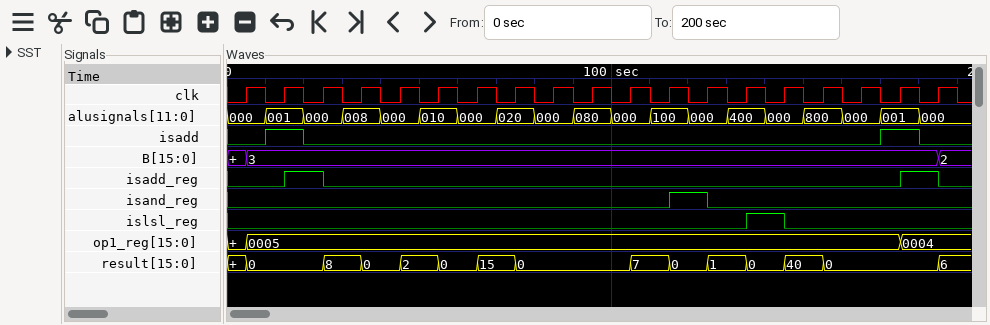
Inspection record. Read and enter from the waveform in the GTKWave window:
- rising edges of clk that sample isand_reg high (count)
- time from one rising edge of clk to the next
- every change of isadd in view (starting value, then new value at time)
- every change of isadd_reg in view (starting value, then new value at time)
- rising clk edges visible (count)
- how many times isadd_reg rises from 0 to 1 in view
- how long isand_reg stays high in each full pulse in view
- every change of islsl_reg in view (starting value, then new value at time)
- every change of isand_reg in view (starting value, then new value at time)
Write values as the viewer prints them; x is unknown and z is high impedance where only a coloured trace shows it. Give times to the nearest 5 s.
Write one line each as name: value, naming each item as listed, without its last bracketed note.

rising edges of clk that sample isand_reg high: 1
time from one rising edge of clk to the next: 10 s
every change of isadd in view: 0, 1 at 10 s, 0 at 20 s, 1 at 170 s, 0 at 180 s
every change of isadd_reg in view: 0, 1 at 15 s, 0 at 25 s, 1 at 175 s, 0 at 185 s
rising clk edges visible: 19
how many times isadd_reg rises from 0 to 1 in view: 2
how long isand_reg stays high in each full pulse in view: 10 s
every change of islsl_reg in view: 0, 1 at 135 s, 0 at 145 s
every change of isand_reg in view: 0, 1 at 115 s, 0 at 125 s
